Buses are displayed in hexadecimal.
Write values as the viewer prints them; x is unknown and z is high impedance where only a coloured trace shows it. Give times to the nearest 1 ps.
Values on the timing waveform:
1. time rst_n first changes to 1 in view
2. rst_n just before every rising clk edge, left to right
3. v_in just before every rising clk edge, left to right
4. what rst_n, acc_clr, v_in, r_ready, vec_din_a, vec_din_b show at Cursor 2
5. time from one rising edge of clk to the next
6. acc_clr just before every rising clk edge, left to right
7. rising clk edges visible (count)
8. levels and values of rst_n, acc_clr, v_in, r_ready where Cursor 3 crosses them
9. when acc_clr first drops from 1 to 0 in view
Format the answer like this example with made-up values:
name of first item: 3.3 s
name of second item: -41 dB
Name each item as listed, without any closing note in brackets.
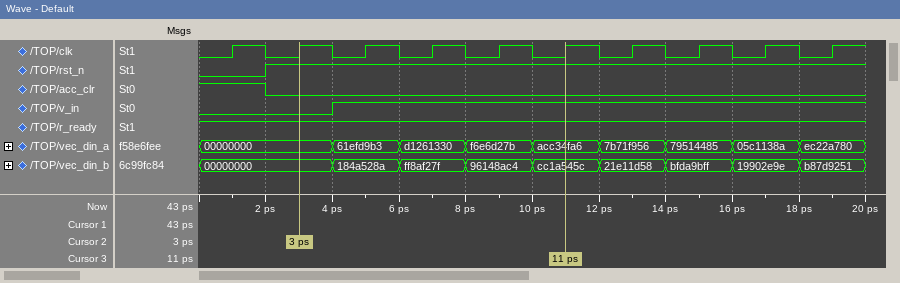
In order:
time rst_n first changes to 1 in view: 2 ps
rst_n just before every rising clk edge, left to right: 0 1 1 1 1 1 1 1 1 1
v_in just before every rising clk edge, left to right: 0 0 1 1 1 1 1 1 1 1
what rst_n, acc_clr, v_in, r_ready, vec_din_a, vec_din_b show at Cursor 2: rst_n=1, acc_clr=0, v_in=0, r_ready=1, vec_din_a=00000000, vec_din_b=00000000
time from one rising edge of clk to the next: 2 ps
acc_clr just before every rising clk edge, left to right: 1 0 0 0 0 0 0 0 0 0
rising clk edges visible: 10
levels and values of rst_n, acc_clr, v_in, r_ready where Cursor 3 crosses them: rst_n=1, acc_clr=0, v_in=1, r_ready=1
when acc_clr first drops from 1 to 0 in view: 2 ps
